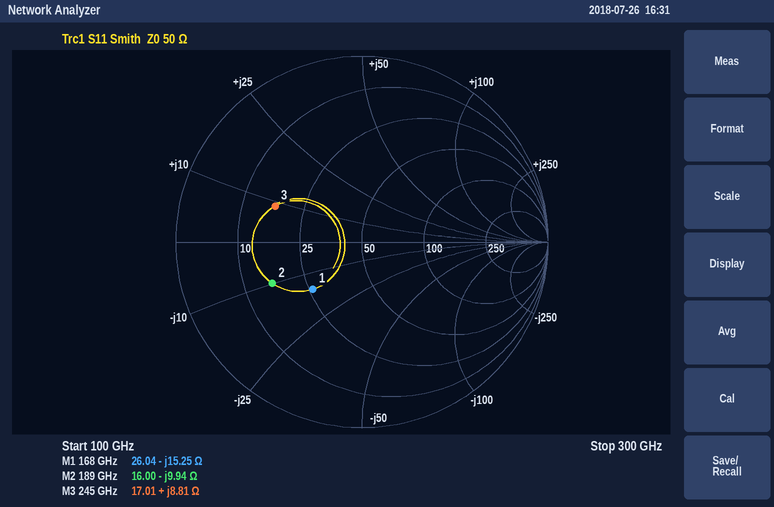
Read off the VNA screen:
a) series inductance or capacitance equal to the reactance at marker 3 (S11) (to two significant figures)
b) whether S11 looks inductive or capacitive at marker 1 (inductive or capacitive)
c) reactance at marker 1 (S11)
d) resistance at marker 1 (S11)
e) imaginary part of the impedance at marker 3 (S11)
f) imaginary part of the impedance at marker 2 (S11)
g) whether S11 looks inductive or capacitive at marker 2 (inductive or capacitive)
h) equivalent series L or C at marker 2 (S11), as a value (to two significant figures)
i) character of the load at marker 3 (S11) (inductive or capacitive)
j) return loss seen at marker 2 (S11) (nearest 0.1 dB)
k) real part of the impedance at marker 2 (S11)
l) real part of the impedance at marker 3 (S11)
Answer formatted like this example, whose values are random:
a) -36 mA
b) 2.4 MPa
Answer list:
a) 5.7 pH
b) capacitive
c) -15.25 Ω
d) 26.04 Ω
e) +8.81 Ω
f) -9.94 Ω
g) capacitive
h) 85 fF
i) inductive
j) 5.5 dB
k) 16.00 Ω
l) 17.01 Ω
